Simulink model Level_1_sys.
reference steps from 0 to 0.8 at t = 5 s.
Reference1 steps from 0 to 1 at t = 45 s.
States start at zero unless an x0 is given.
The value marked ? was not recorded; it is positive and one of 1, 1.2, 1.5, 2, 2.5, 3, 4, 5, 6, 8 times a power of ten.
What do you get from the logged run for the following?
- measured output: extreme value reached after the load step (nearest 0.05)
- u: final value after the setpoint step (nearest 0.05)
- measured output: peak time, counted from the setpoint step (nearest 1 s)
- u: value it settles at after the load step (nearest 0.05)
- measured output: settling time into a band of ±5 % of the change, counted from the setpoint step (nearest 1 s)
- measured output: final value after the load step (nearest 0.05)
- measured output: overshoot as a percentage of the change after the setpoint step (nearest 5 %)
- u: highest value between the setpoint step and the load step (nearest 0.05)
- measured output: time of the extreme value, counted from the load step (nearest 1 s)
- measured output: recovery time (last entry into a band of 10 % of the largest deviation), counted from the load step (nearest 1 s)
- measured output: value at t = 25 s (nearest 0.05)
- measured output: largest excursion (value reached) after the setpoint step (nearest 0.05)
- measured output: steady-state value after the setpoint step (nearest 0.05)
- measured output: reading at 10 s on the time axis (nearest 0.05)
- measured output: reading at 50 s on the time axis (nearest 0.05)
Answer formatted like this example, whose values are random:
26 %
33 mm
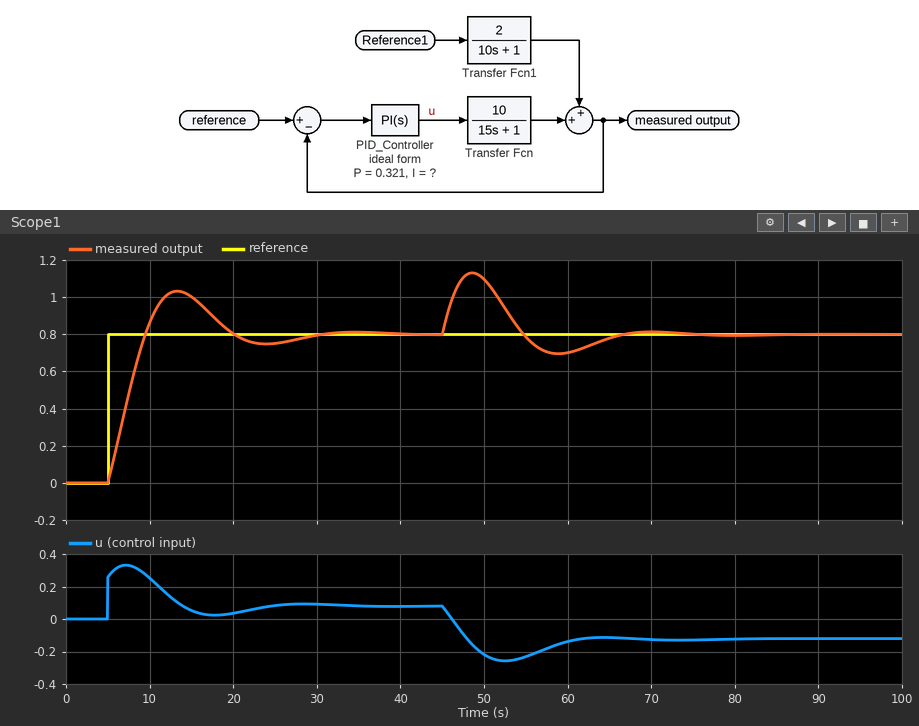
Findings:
1.15
0.10
8 s
-0.10
21 s
0.80
30 %
0.35
4 s
19 s
0.75
1.05
0.80
0.85
1.10
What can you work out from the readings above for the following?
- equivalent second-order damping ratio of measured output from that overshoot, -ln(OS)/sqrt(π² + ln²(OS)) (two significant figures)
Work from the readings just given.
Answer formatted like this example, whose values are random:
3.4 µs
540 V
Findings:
0.36
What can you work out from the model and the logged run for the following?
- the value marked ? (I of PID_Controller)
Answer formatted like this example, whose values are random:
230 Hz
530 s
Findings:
0.5
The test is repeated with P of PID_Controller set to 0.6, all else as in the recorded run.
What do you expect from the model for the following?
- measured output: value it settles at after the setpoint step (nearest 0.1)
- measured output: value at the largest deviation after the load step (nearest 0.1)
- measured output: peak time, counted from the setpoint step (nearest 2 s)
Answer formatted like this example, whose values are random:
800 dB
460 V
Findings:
0.8
1.0
6 s
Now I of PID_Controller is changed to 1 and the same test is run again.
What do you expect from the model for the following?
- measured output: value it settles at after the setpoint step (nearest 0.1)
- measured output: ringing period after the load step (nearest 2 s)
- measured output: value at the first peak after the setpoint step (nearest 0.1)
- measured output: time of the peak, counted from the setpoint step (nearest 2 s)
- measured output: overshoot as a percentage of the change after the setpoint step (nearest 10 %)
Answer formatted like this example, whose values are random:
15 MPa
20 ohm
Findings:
0.8
14 s
1.1
6 s
40 %
